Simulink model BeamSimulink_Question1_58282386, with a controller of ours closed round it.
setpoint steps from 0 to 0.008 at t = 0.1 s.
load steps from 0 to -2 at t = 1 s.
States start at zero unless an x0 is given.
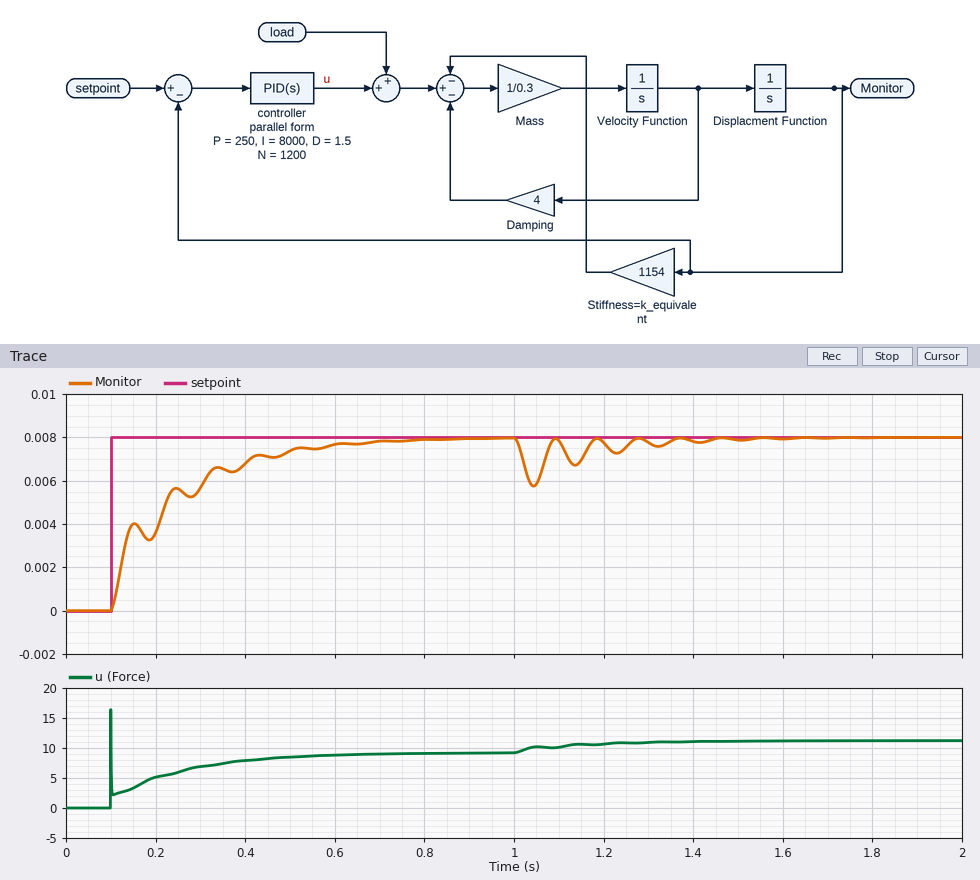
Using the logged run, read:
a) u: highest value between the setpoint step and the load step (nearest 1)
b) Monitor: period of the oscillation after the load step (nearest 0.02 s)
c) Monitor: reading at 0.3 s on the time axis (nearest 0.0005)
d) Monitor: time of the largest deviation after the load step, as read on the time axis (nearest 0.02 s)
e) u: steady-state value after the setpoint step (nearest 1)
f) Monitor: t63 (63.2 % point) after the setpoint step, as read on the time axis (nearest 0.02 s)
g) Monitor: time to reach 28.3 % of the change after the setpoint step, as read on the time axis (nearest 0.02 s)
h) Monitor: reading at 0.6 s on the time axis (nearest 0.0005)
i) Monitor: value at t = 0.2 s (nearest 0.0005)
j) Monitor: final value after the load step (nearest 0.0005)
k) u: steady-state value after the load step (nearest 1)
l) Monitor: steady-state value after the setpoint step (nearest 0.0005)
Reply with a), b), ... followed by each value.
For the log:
a) 16
b) 0.10 s
c) 0.0055
d) 1.04 s
e) 9
f) 0.22 s
g) 0.12 s
h) 0.0075
i) 0.0035
j) 0.0080
k) 11
l) 0.0080
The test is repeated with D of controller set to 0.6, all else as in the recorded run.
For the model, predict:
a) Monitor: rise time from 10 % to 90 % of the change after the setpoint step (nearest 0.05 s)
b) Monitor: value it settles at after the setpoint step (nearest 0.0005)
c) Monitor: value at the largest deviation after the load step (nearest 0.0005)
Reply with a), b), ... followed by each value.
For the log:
a) 0.30 s
b) 0.0080
c) 0.0055
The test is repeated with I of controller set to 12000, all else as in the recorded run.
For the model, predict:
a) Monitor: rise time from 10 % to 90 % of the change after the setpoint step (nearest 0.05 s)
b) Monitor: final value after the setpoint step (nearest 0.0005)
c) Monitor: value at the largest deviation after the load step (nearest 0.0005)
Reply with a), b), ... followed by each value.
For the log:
a) 0.20 s
b) 0.0080
c) 0.0060
